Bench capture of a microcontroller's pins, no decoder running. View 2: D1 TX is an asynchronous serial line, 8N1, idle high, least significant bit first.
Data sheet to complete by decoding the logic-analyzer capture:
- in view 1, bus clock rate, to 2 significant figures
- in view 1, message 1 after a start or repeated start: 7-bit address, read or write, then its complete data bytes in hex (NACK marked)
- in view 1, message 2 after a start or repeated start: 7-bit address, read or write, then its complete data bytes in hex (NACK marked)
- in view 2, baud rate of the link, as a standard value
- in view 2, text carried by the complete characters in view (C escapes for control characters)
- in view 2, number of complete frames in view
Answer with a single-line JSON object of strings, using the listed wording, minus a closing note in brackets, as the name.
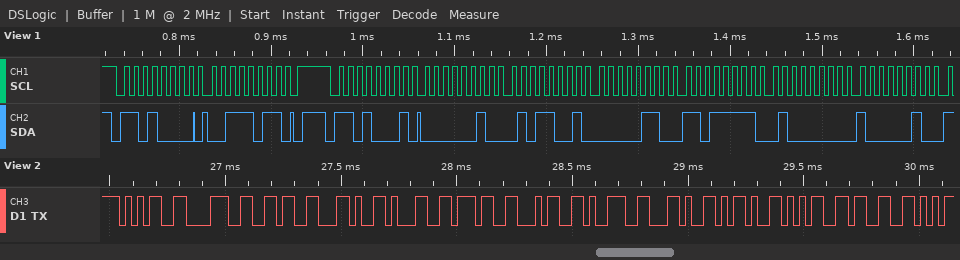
{"in view 1, bus clock rate, to 2 significant figures": "100 kHz", "in view 1, message 1 after a start or repeated start: 7-bit address, read or write, then its complete data bytes in hex": "0x68 write: 3B", "in view 1, message 2 after a start or repeated start: 7-bit address, read or write, then its complete data bytes in hex": "0x68 read: 02 59 06 DF 40 82", "in view 2, baud rate of the link, as a standard value": "38400 baud", "in view 2, text carried by the complete characters in view": "\"586,1749,-53\"", "in view 2, number of complete frames in view": "12"}
